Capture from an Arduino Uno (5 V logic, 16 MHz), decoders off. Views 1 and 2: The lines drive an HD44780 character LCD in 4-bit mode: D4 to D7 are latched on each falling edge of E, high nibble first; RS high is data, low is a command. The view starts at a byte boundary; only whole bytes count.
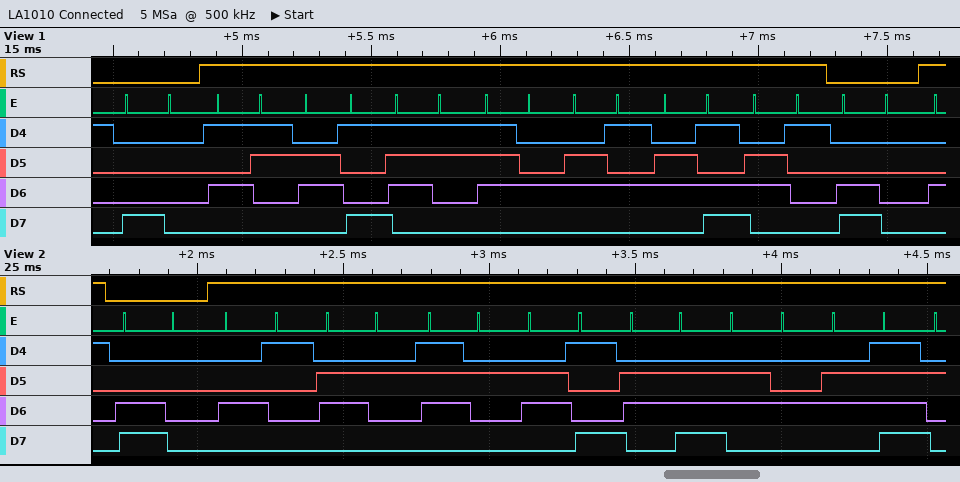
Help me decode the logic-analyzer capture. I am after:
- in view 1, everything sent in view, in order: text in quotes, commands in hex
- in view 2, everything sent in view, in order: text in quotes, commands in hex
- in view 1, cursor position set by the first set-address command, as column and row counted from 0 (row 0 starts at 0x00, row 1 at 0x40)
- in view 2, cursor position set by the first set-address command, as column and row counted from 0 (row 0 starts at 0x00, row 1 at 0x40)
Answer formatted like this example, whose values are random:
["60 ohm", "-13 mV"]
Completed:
["0x80 \"Sistema\" 0xC0", "0xC0 \"Abrindo\"", "column 0, row 0", "column 0, row 1"]
